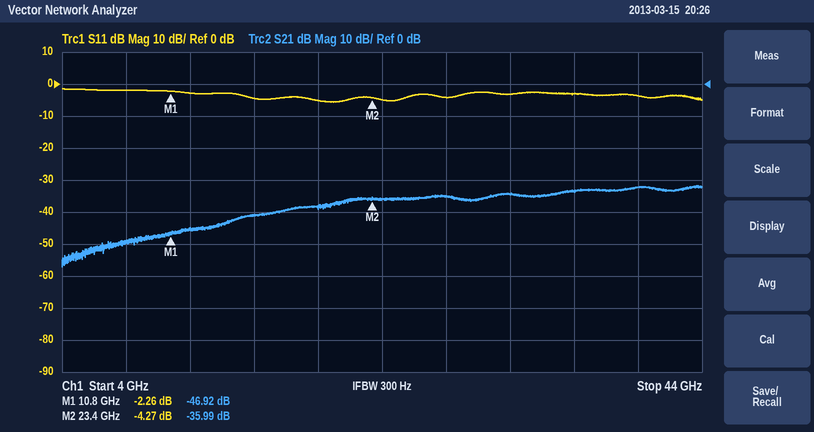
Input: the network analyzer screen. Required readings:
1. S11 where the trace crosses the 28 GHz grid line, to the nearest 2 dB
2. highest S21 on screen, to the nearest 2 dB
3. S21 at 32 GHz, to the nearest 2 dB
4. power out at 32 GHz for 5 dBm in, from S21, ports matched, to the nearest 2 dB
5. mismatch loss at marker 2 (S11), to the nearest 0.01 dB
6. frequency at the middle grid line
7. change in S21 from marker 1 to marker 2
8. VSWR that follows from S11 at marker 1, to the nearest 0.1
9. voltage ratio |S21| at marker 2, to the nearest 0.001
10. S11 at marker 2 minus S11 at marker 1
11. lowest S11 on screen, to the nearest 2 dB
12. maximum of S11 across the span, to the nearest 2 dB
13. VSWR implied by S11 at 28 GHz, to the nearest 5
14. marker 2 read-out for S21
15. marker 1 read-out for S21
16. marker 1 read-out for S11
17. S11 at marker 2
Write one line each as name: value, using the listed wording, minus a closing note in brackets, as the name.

S11 where the trace crosses the 28 GHz grid line, to the nearest 2 dB: -4 dB
highest S21 on screen, to the nearest 2 dB: -32 dB
S21 at 32 GHz, to the nearest 2 dB: -34 dB
power out at 32 GHz for 5 dBm in, from S21, ports matched, to the nearest 2 dB: -30 dBm
mismatch loss at marker 2 (S11), to the nearest 0.01 dB: 2.04 dB
frequency at the middle grid line: 24 GHz
change in S21 from marker 1 to marker 2: 10.93 dB
VSWR that follows from S11 at marker 1, to the nearest 0.1: 7.7
voltage ratio |S21| at marker 2, to the nearest 0.001: 0.016
S11 at marker 2 minus S11 at marker 1: -2.01 dB
lowest S11 on screen, to the nearest 2 dB: -6 dB
maximum of S11 across the span, to the nearest 2 dB: -2 dB
VSWR implied by S11 at 28 GHz, to the nearest 5: 5
marker 2 read-out for S21: -35.99 dB
marker 1 read-out for S21: -46.92 dB
marker 1 read-out for S11: -2.26 dB
S11 at marker 2: -4.27 dB
